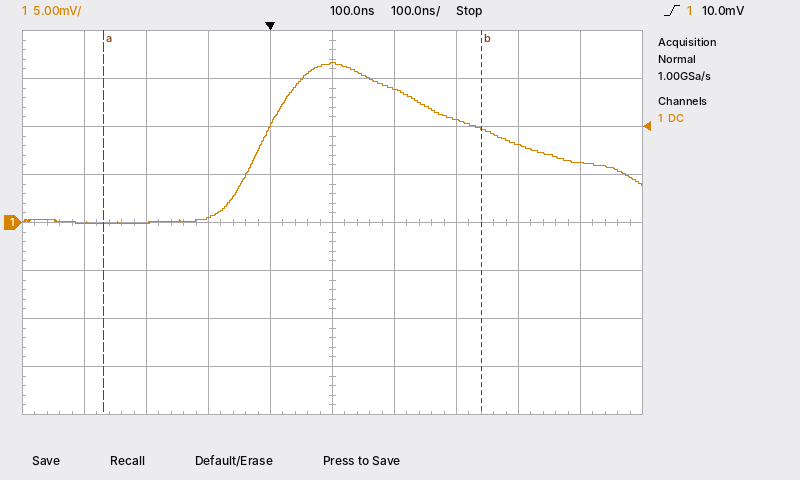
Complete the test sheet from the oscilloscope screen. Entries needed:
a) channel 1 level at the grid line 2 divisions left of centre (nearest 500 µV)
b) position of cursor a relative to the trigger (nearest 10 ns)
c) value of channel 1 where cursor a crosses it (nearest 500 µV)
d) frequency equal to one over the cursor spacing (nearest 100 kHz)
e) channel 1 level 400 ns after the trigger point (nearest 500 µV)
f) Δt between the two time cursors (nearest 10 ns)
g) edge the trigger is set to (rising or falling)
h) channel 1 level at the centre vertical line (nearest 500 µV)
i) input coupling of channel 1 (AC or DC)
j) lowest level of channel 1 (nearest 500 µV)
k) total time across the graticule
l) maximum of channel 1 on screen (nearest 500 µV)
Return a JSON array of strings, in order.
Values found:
["500 µV", "-270 ns", "0.0 mV", "1.6 MHz", "8.0 mV", "610 ns", "rising", "16.5 mV", "DC", "0.0 mV", "1 µs", "16.5 mV"]
